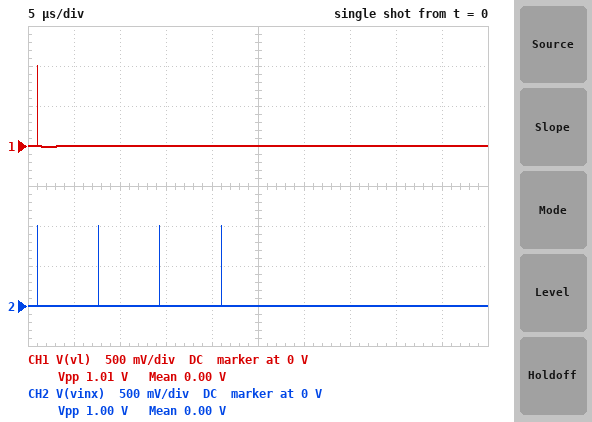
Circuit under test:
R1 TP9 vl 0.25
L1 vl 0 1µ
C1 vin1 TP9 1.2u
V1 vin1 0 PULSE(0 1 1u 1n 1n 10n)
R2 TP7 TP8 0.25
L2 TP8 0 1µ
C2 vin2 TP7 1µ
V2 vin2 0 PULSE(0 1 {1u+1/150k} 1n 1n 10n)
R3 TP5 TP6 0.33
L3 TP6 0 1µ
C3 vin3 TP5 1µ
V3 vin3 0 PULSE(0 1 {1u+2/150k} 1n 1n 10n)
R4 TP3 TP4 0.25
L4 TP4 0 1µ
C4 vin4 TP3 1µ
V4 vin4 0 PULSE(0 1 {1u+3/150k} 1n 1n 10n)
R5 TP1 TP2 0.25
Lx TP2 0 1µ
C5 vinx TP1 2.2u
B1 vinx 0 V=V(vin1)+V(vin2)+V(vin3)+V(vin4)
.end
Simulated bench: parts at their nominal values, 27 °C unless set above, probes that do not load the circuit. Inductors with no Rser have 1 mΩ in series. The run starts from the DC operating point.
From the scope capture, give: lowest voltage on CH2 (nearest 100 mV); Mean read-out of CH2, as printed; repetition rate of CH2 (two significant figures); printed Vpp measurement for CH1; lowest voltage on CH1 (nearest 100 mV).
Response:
0 V
0.00 V
150 kHz
1.01 V
0 V
